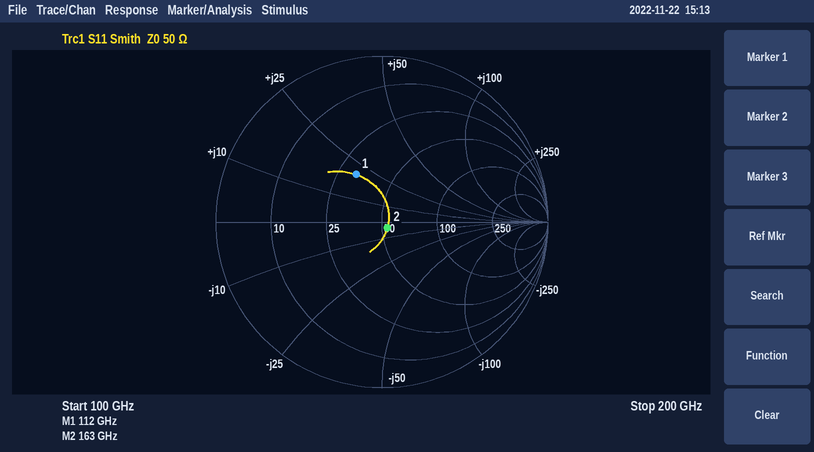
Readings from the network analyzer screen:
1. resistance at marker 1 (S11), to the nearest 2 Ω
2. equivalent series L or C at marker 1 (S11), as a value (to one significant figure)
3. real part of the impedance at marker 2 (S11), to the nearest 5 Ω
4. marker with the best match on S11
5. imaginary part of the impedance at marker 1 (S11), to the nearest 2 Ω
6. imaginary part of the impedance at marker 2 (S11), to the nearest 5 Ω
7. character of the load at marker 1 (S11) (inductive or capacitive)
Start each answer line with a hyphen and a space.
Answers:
- 32 Ω
- 30 pH
- 55 Ω
- marker 2
- +20 Ω
- -5 Ω
- inductive
